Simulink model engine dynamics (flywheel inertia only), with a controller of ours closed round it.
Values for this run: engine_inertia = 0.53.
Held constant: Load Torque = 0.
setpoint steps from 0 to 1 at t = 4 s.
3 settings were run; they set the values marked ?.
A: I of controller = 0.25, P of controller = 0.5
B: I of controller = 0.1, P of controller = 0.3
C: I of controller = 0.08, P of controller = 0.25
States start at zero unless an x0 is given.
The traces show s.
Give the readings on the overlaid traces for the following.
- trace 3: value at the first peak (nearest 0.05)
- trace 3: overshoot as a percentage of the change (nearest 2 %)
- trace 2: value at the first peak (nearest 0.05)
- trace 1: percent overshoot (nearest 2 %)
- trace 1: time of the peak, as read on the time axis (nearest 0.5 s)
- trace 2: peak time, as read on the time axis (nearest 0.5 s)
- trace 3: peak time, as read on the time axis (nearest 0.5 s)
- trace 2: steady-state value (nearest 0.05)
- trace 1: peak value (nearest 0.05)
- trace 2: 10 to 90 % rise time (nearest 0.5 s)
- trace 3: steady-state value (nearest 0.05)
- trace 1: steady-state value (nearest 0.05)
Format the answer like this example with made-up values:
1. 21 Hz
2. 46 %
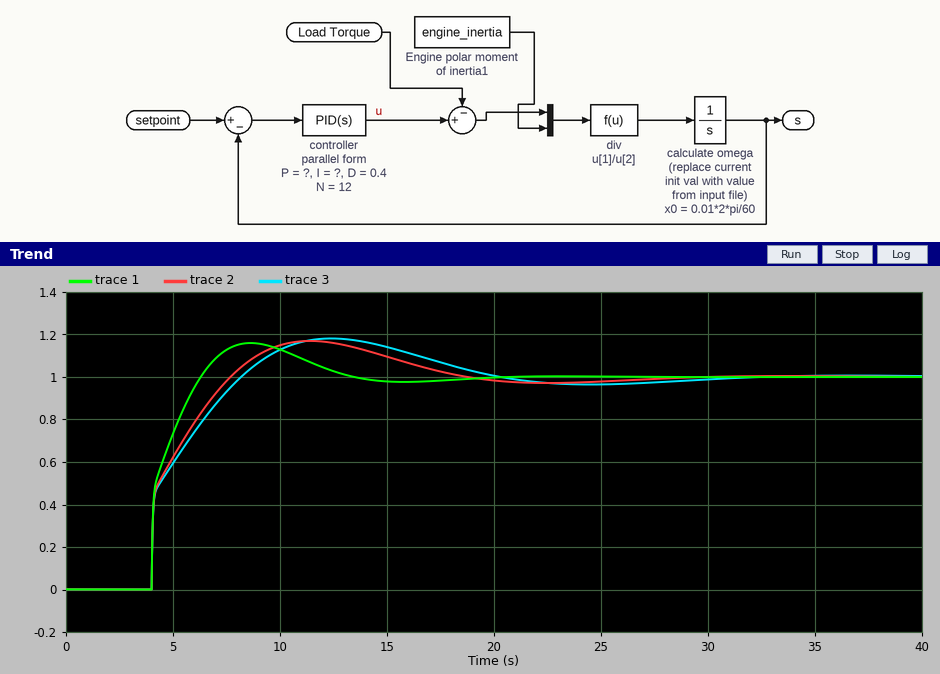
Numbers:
1. 1.20
2. 18 %
3. 1.15
4. 16 %
5. 8.5 s
6. 11.5 s
7. 12.5 s
8. 1.00
9. 1.15
10. 3.0 s
11. 1.00
12. 1.00
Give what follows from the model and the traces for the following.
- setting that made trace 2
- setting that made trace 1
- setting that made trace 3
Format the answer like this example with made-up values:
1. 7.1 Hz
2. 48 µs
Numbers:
1. B
2. A
3. C
